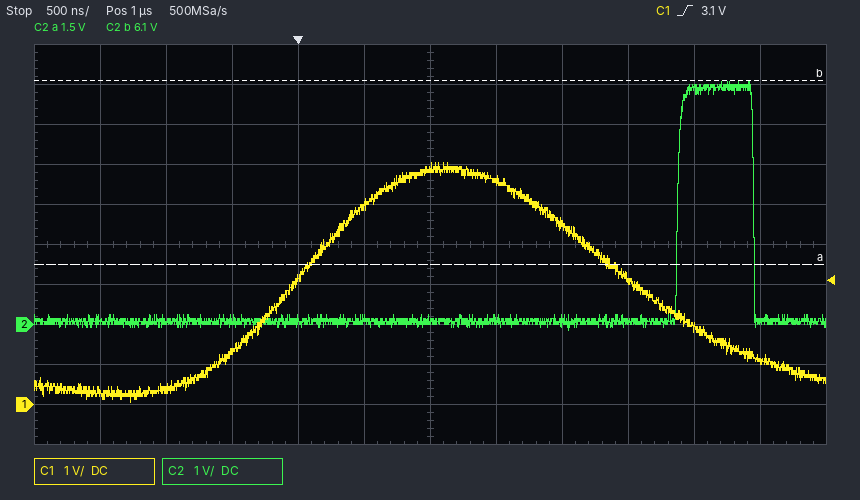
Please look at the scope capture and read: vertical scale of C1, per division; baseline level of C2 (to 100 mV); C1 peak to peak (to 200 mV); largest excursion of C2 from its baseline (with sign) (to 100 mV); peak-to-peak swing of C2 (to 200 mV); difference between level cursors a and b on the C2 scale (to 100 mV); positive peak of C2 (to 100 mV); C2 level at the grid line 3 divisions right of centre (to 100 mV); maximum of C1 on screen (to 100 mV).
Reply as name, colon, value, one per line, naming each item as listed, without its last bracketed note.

vertical scale of C1, per division: 1 V
baseline level of C2: 100 mV
C1 peak to peak: 6.0 V
largest excursion of C2 from its baseline (with sign): +6.0 V
peak-to-peak swing of C2: 6.2 V
difference between level cursors a and b on the C2 scale: 4.6 V
positive peak of C2: 6.1 V
C2 level at the grid line 3 divisions right of centre: 100 mV
maximum of C1 on screen: 6.0 V
